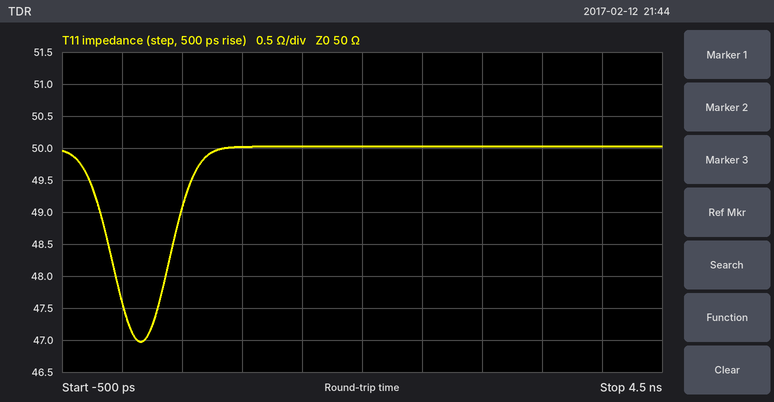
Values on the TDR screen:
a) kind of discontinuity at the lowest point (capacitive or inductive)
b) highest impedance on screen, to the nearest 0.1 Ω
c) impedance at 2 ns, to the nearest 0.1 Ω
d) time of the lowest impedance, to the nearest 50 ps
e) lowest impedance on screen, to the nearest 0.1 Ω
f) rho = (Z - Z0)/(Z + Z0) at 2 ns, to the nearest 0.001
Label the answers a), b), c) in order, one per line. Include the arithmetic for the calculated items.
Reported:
a) capacitive
b) 50.0 Ω
c) 50.0 Ω
d) 150 ps
e) 47.0 Ω
f) (50 − 50)/(50 + 50) ≈ 0.000
